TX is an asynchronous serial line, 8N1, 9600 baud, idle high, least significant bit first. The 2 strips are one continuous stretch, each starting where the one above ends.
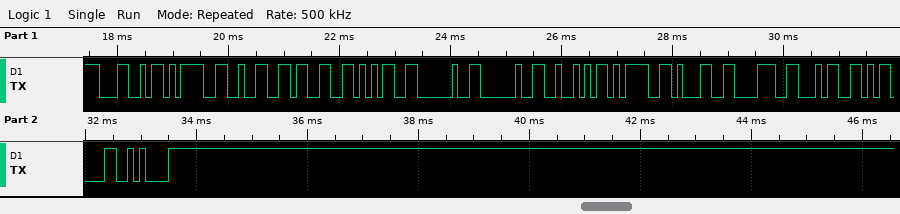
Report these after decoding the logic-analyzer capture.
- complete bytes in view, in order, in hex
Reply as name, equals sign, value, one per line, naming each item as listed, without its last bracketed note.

complete bytes in view, in order, in hex = 0x4C 0x3D 0x32 0x33 0x35 0x20 0x20 0x52 0x3D 0x31 0x38 0x34 0x0D 0x0A
